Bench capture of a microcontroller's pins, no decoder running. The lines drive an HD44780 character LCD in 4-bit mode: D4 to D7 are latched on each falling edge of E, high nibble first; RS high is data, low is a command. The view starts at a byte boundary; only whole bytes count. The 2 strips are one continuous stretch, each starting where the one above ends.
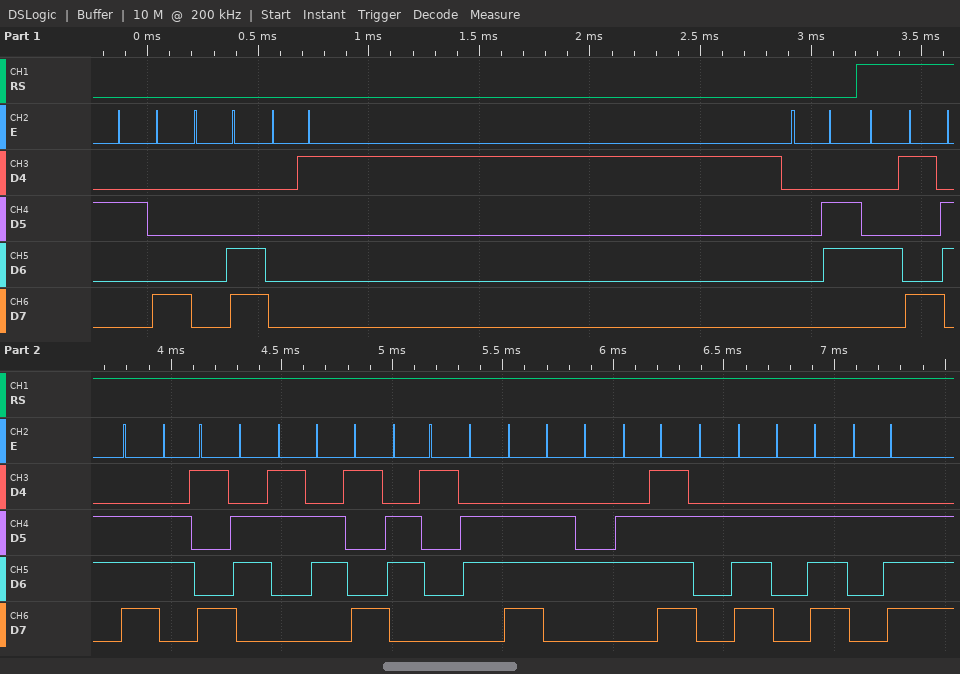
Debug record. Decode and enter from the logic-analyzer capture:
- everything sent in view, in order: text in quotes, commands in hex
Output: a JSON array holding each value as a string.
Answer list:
["0x28 0x0C 0x01 0x06 \"Iniciando...\""]
